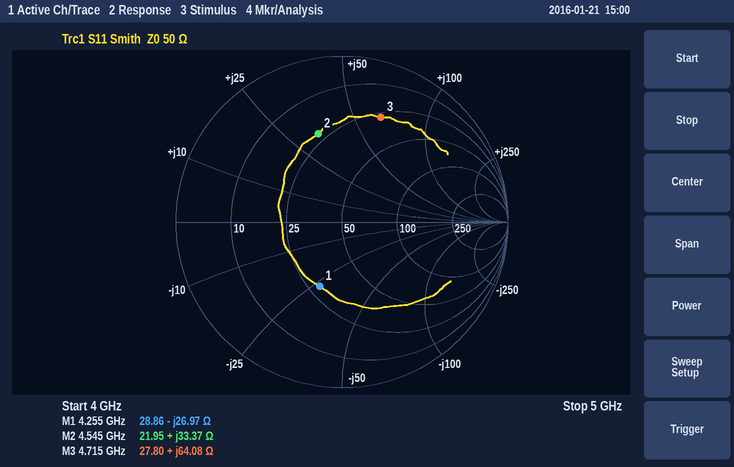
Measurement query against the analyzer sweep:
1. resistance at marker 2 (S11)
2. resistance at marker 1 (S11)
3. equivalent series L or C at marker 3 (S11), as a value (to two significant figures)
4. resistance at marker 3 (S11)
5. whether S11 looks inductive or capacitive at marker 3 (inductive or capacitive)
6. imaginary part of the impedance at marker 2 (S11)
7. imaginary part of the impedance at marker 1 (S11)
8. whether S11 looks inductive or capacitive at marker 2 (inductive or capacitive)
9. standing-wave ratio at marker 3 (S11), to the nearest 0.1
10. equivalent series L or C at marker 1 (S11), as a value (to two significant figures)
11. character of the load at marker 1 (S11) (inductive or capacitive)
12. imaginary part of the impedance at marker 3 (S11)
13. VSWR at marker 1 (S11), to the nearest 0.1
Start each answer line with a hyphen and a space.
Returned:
- 21.95 Ω
- 28.86 Ω
- 2.2 nH
- 27.80 Ω
- inductive
- +33.37 Ω
- -26.97 Ω
- inductive
- 5.1
- 1.4 pF
- capacitive
- +64.08 Ω
- 2.4
